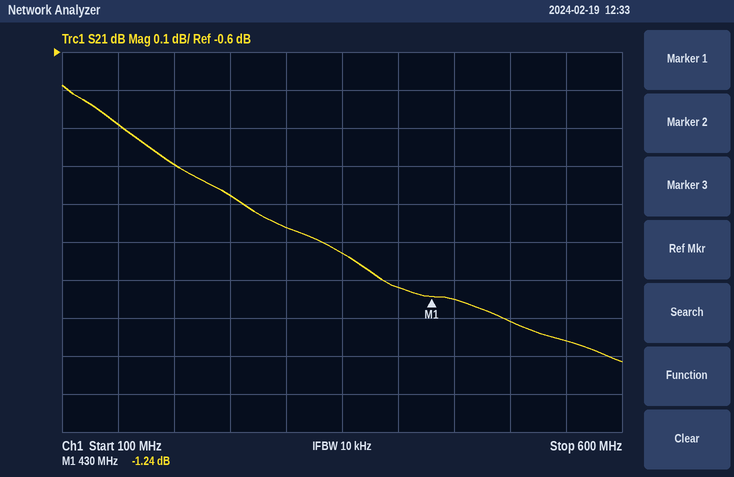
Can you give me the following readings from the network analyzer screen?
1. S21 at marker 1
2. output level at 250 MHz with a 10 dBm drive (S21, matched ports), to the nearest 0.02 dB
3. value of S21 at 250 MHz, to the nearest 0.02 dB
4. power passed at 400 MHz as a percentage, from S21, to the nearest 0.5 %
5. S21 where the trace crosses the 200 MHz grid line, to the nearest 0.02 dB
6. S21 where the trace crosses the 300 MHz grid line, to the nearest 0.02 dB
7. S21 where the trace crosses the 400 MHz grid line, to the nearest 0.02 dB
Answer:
-1.24 dB
9.02 dBm
-0.98 dB
75.5 %
-0.90 dB
-1.06 dB
-1.22 dB
